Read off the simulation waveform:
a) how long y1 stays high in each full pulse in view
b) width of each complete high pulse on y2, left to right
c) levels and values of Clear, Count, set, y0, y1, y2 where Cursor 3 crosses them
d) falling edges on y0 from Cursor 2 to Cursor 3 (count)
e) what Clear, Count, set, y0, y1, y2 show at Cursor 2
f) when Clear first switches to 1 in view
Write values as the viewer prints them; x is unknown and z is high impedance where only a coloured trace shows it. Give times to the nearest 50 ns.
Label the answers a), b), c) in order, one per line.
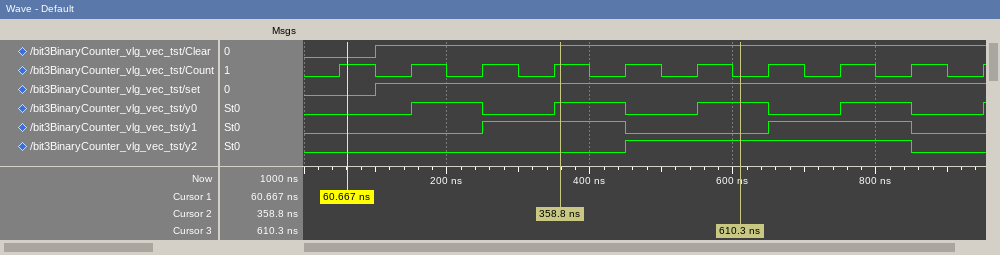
a) 200 ns, 200 ns
b) 400 ns
c) Clear=1, Count=0, set=1, y0=1, y1=0, y2=1
d) 1
e) Clear=1, Count=1, set=1, y0=1, y1=1, y2=0
f) 100 ns
